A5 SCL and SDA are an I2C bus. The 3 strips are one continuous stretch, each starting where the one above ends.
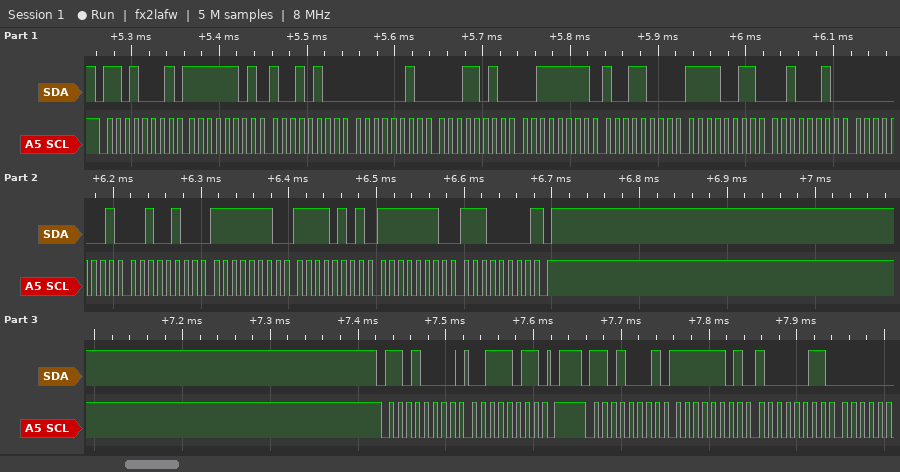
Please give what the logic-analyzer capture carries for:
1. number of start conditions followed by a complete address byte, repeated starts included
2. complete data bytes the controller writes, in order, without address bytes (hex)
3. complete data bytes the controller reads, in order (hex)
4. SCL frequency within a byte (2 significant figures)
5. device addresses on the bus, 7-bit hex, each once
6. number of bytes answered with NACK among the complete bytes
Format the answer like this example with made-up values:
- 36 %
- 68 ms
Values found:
- 3
- 3B
- FD 94 02 1A 3F 98 F3 22 01 24 FE F5 FE E0 FD 83
- 100 kHz
- 0x68
- 1
